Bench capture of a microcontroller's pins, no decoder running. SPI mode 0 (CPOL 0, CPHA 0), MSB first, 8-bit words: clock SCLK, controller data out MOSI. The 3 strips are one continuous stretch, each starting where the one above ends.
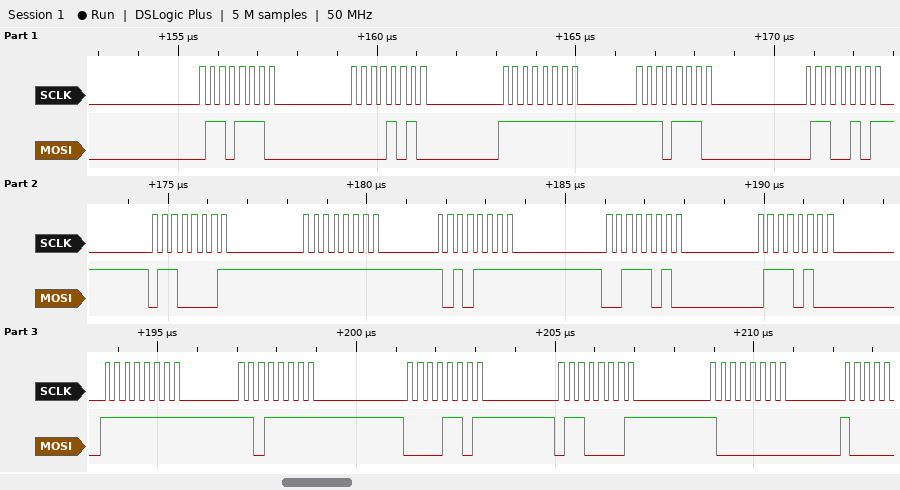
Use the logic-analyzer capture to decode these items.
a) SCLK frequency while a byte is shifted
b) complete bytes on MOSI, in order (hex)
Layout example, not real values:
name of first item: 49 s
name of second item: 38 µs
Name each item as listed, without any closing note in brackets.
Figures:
SCLK frequency while a byte is shifted: 4 MHz
complete bytes on MOSI, in order: 6E 0A FF EE 65 61 FF AF 3A 74 FF DF 0D 61 80
